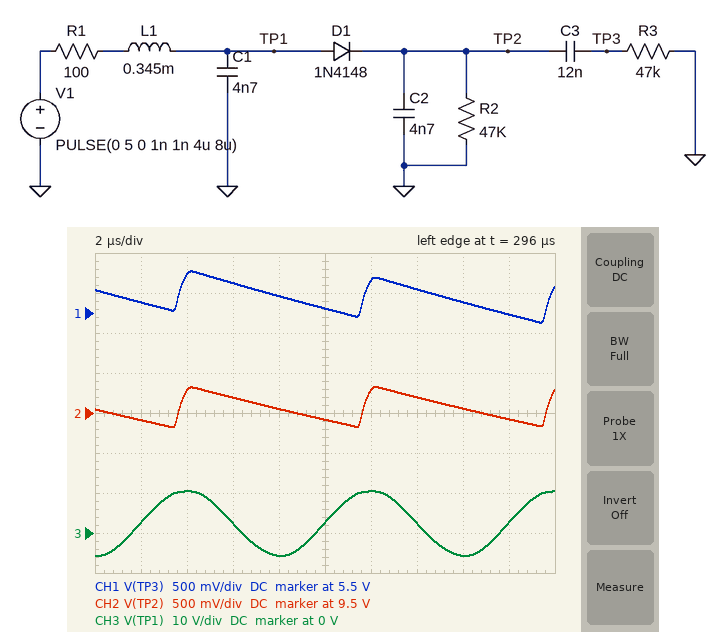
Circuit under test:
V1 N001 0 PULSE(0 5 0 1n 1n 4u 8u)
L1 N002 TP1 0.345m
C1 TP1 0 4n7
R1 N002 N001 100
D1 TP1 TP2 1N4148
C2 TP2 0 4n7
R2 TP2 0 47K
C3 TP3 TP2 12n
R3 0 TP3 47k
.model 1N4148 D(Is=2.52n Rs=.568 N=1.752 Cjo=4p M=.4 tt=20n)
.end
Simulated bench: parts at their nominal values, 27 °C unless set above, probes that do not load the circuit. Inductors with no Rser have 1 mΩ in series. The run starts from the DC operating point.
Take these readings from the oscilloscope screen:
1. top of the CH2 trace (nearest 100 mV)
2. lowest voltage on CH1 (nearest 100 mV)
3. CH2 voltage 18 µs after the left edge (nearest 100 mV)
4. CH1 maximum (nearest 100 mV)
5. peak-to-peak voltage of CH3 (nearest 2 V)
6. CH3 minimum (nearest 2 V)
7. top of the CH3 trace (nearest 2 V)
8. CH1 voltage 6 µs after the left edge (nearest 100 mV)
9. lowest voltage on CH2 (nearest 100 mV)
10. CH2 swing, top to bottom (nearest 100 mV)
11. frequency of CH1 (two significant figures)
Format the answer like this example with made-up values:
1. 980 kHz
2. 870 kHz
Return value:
1. 9.8 V
2. 5.4 V
3. 9.4 V
4. 6.0 V
5. 16 V
6. -6 V
7. 10 V
8. 5.9 V
9. 9.3 V
10. 500 mV
11. 120 kHz
